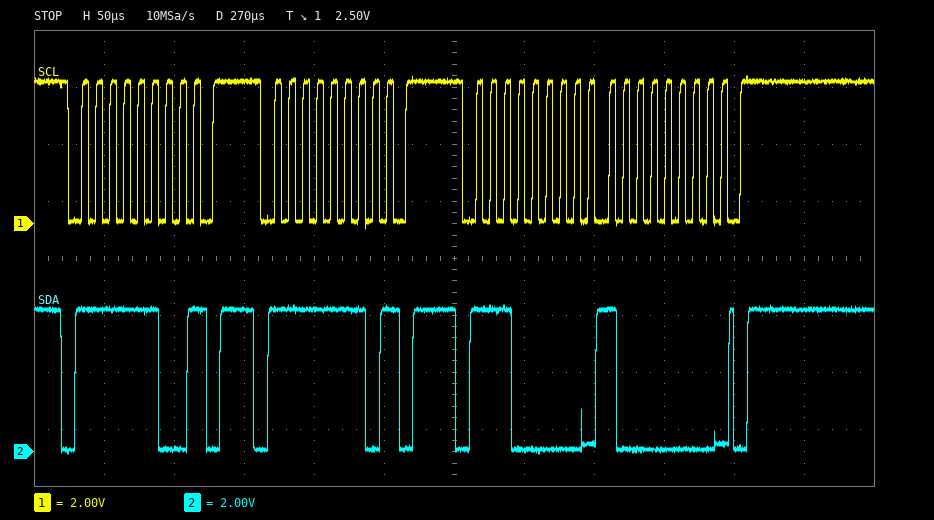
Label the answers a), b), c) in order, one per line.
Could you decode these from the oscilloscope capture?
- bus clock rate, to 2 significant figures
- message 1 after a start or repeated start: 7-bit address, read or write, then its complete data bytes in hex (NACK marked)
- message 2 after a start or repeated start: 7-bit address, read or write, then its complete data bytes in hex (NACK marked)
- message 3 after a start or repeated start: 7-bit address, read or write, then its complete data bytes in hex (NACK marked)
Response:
a) 100 kHz
b) 0x7E write NACK
c) 0x7F write NACK
d) 0x70 write: 80
